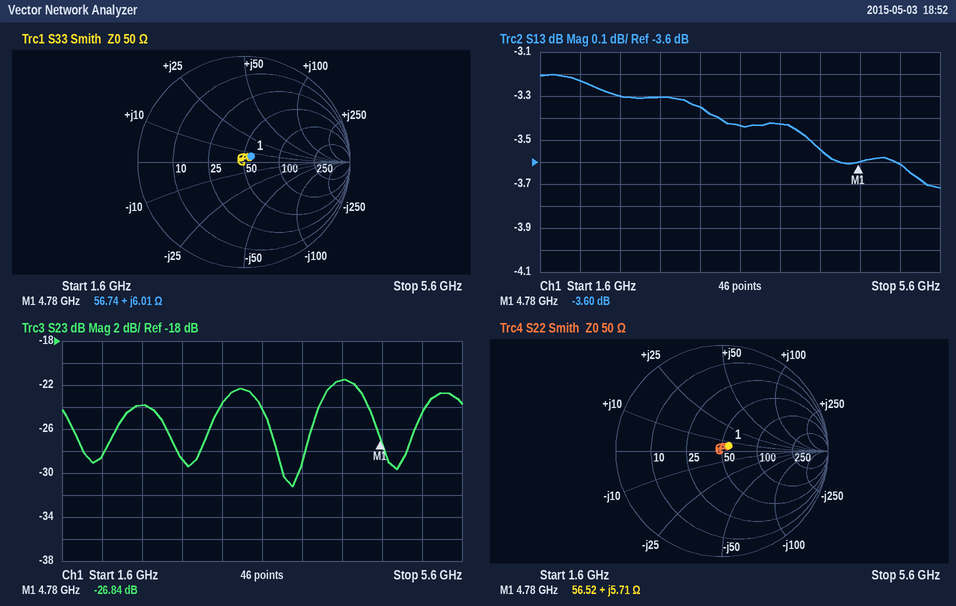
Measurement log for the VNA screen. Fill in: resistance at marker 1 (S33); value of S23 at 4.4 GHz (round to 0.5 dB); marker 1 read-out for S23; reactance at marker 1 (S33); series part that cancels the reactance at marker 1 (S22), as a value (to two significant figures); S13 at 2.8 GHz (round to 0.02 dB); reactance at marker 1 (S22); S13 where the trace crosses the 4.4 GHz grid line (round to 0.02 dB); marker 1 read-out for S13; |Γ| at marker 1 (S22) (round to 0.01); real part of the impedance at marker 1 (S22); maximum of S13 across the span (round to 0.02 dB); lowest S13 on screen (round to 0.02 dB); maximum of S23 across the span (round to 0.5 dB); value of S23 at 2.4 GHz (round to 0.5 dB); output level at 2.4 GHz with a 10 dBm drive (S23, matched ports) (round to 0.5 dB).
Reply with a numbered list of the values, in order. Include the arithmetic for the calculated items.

1. 56.74 Ω
2. -21.5 dB
3. -26.84 dB
4. +6.01 Ω
5. C = 1/(2π × 4.78 GHz × 5.71 Ω) ≈ 5.8 pF
6. -3.30 dB
7. +5.71 Ω
8. -3.54 dB
9. -3.60 dB
10. 0.08
11. 56.52 Ω
12. -3.20 dB
13. -3.72 dB
14. -21.5 dB
15. -24.0 dB
16. 10 dBm + (-24.0 dB) = -14.0 dBm
